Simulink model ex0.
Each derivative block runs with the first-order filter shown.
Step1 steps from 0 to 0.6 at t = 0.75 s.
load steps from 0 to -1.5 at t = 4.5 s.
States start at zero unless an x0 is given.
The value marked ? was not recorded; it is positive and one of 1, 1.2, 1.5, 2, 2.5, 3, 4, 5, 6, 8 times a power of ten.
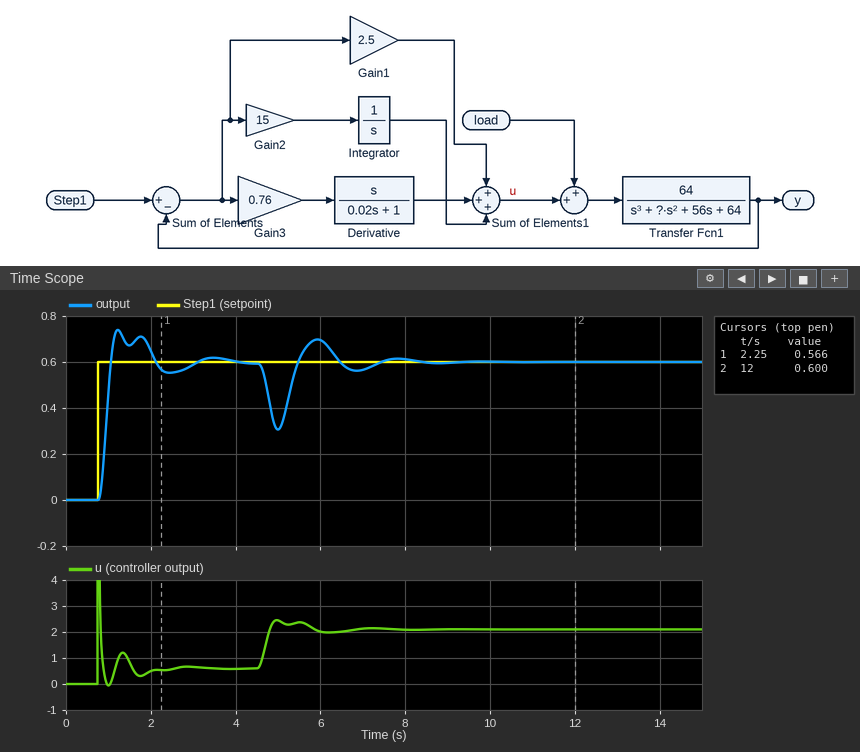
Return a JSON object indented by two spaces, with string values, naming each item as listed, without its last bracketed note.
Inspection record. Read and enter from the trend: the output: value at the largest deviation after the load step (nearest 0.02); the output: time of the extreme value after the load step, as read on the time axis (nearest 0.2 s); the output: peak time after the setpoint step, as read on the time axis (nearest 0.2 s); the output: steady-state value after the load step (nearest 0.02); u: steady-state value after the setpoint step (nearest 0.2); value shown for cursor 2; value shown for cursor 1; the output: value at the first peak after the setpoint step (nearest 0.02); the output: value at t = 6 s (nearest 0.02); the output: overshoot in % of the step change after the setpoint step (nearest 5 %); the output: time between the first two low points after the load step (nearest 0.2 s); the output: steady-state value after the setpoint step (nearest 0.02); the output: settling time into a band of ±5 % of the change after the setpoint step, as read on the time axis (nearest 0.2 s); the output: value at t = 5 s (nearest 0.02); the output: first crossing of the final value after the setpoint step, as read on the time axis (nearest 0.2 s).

{
  "the output: value at the largest deviation after the load step": "0.30",
  "the output: time of the extreme value after the load step, as read on the time axis": "5.0 s",
  "the output: peak time after the setpoint step, as read on the time axis": "1.2 s",
  "the output: steady-state value after the load step": "0.60",
  "u: steady-state value after the setpoint step": "0.6",
  "value shown for cursor 2": "0.600",
  "value shown for cursor 1": "0.566",
  "the output: value at the first peak after the setpoint step": "0.74",
  "the output: value at t = 6 s": "0.70",
  "the output: overshoot in % of the step change after the setpoint step": "25 %",
  "the output: time between the first two low points after the load step": "1.8 s",
  "the output: steady-state value after the setpoint step": "0.60",
  "the output: settling time into a band of ±5 % of the change after the setpoint step, as read on the time axis": "2.8 s",
  "the output: value at t = 5 s": "0.30",
  "the output: first crossing of the final value after the setpoint step, as read on the time axis": "1.0 s"
}
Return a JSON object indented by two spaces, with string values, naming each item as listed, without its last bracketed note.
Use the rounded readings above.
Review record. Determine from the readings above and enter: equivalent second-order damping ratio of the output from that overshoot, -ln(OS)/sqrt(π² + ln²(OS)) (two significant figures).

{
  "equivalent second-order damping ratio of the output from that overshoot, -ln(OS)/sqrt(π² + ln²(OS))": "0.40"
}
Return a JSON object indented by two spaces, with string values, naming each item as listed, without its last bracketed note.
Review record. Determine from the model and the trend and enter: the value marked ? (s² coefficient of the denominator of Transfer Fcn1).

{
  "the value marked ?": "8"
}
